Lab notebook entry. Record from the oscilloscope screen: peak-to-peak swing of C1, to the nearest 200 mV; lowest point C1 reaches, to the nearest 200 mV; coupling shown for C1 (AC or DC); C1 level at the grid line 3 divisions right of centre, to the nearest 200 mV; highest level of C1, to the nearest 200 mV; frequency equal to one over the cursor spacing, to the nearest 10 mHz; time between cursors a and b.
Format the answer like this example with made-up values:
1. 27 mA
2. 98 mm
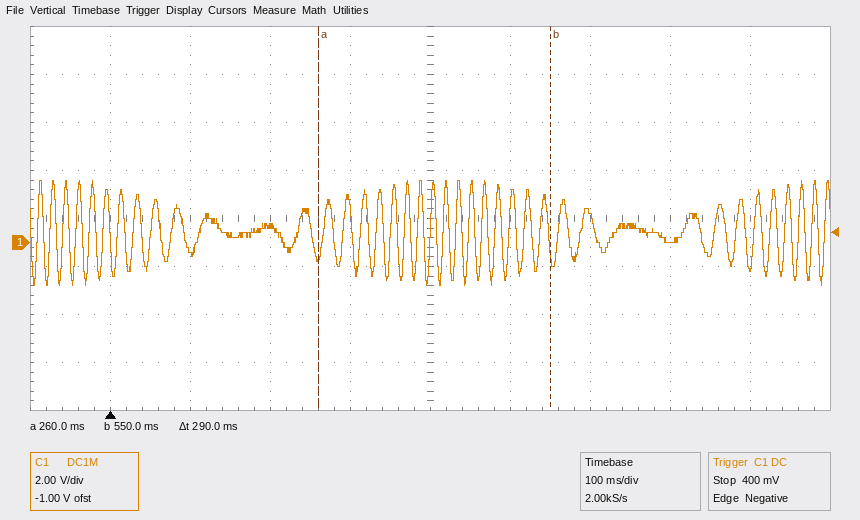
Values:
1. 4.4 V
2. -1.8 V
3. DC
4. 0.0 V
5. 2.6 V
6. 3.45 Hz
7. 290 ms
